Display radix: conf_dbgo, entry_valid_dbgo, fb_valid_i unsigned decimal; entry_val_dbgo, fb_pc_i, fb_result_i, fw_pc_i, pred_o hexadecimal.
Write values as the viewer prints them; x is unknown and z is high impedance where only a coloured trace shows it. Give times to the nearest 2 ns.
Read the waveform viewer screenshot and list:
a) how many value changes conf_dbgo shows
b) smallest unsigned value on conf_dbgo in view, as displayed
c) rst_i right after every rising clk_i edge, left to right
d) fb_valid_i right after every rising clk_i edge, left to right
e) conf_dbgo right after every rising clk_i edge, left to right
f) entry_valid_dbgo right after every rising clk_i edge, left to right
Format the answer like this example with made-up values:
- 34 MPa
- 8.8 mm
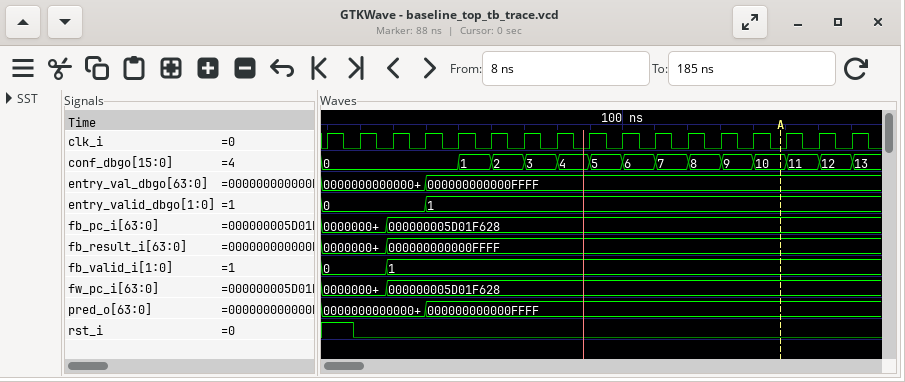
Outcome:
- 13
- 0
- 1 0 0 0 0 0 0 0 0 0 0 0 0 0 0 0 0
- 0, 0, 1, 1, 1, 1, 1, 1, 1, 1, 1, 1, 1, 1, 1, 1, 1
- 0, 0, 0, 0, 1, 2, 3, 4, 5, 6, 7, 8, 9, 10, 11, 12, 13
- 0, 0, 0, 1, 1, 1, 1, 1, 1, 1, 1, 1, 1, 1, 1, 1, 1
